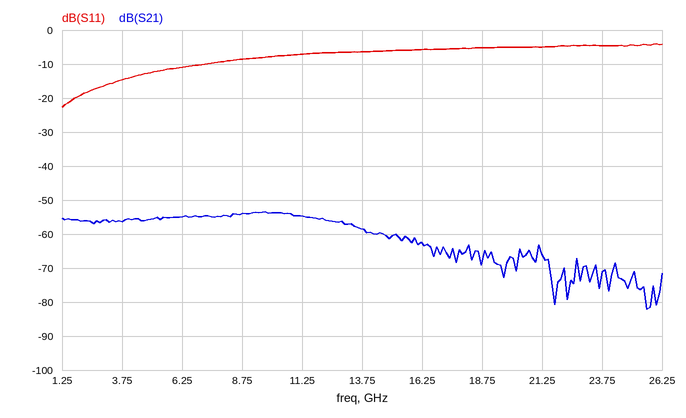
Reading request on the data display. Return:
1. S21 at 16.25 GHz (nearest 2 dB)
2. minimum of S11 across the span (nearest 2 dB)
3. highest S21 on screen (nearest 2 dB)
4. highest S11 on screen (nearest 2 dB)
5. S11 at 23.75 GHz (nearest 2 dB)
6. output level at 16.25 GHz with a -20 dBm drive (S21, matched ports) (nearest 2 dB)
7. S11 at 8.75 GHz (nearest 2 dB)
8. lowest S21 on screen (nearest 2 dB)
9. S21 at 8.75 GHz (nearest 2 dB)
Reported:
-62 dB
-22 dB
-54 dB
-4 dB
-4 dB
-82 dBm
-8 dB
-82 dB
-54 dB
